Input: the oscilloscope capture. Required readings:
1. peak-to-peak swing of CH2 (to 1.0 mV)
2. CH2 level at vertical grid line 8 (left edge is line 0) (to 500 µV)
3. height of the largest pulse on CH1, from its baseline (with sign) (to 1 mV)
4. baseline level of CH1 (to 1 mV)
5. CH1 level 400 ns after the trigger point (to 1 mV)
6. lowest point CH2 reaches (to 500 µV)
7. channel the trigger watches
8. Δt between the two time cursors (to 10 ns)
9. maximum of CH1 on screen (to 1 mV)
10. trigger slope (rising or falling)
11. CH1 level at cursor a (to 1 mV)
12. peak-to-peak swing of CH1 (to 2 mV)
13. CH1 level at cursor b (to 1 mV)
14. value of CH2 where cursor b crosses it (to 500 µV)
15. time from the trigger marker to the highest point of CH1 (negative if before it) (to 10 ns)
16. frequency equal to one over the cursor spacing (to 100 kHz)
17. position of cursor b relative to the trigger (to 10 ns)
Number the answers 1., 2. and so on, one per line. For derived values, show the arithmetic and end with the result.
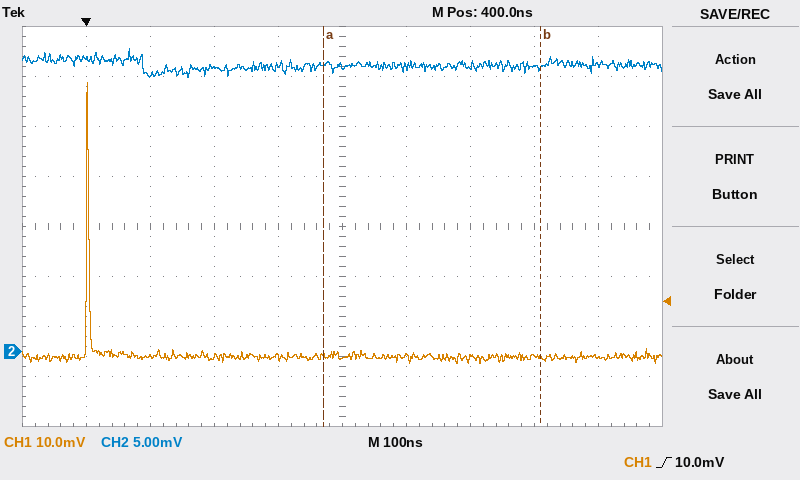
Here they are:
1. 3.0 mV
2. 28.5 mV
3. 54 mV − (-1 mV) = +55 mV
4. -1 mV
5. -1 mV
6. 27.5 mV
7. CH1
8. 340 ns
9. 54 mV
10. rising
11. -1 mV
12. 56 mV
13. -1 mV
14. 28.5 mV
15. 0 ns
16. 1 / 340 ns ≈ 2.9 MHz
17. +710 ns
